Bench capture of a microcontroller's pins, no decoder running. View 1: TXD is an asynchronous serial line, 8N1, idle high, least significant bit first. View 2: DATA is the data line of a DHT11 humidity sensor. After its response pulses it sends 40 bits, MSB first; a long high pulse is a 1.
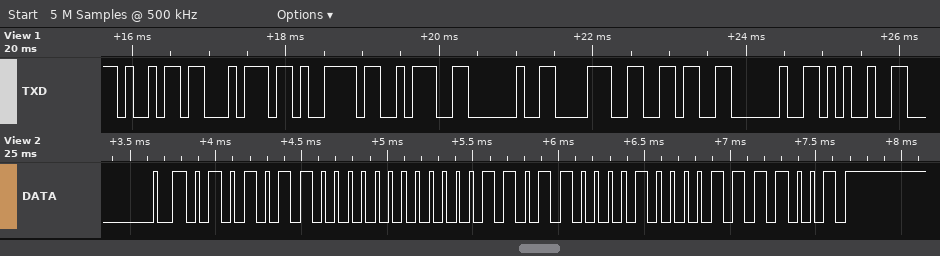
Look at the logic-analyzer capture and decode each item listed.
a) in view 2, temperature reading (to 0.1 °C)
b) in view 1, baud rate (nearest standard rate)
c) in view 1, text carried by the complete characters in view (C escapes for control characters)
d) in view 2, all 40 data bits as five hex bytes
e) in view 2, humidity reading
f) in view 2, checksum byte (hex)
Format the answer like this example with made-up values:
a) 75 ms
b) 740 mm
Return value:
a) 27.8 °C
b) 9600 baud
c) "ity: 86 %"
d) 56 00 1B 08 79
e) 86 %
f) 0x79
